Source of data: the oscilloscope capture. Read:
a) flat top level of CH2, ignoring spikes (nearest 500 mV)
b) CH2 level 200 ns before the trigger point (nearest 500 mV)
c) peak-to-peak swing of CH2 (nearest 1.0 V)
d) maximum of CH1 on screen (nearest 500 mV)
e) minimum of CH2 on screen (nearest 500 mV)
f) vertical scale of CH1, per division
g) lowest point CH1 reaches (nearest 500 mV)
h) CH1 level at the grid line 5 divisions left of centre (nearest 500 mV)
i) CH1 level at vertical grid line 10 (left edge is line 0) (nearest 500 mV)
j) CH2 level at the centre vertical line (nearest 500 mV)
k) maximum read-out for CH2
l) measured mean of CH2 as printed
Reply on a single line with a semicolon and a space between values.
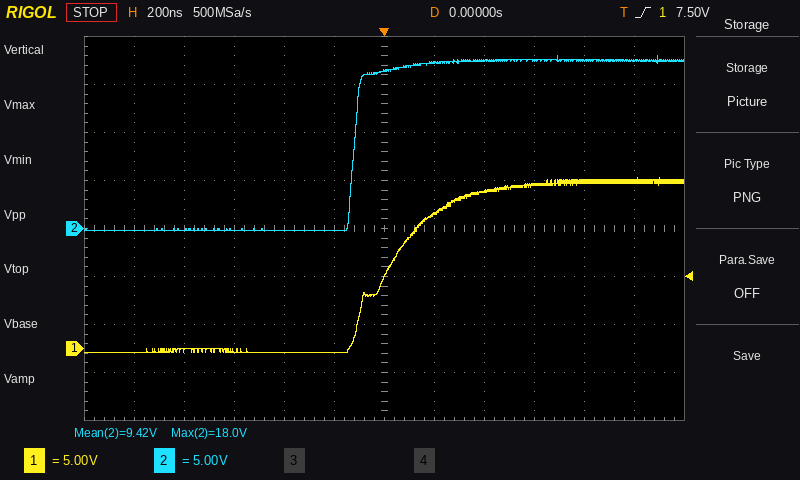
17.5 V; 0.0 V; 18.0 V; 18.0 V; 0.0 V; 5 V; -500 mV; -500 mV; 17.5 V; 16.5 V; 18.0 V; 9.42 V
